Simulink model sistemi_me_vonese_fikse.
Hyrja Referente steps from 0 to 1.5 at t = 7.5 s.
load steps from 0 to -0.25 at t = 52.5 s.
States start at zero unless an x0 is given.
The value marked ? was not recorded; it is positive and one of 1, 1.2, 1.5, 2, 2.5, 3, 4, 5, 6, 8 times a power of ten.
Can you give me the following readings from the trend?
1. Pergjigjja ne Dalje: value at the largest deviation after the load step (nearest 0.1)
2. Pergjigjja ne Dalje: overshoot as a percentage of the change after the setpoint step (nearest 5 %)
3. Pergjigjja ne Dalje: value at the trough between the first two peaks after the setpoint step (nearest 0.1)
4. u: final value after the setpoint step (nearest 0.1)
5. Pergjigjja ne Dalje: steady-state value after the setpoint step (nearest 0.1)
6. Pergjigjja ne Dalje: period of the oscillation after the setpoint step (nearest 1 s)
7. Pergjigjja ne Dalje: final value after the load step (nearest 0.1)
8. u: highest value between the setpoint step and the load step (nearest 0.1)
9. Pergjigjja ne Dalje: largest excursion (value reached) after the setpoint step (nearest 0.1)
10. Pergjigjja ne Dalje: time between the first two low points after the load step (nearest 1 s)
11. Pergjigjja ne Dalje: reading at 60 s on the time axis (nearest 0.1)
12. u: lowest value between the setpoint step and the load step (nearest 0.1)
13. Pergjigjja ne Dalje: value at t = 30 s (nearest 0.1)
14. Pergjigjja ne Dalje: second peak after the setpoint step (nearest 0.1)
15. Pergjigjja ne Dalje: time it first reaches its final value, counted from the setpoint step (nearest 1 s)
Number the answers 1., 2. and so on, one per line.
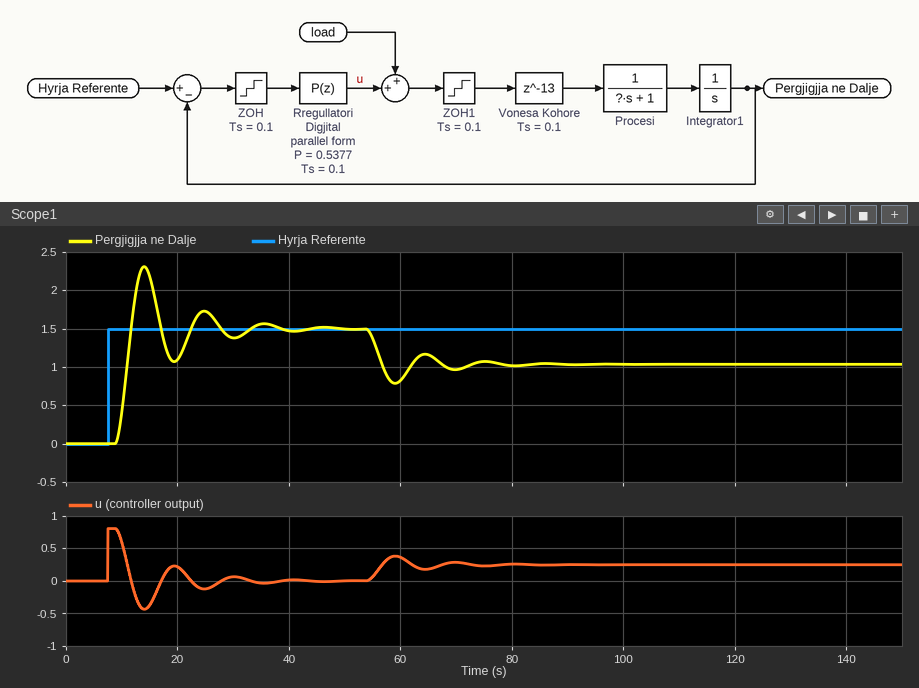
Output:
1. 0.8
2. 55 %
3. 1.1
4. 0.0
5. 1.5
6. 11 s
7. 1.0
8. 0.8
9. 2.3
10. 11 s
11. 0.8
12. -0.4
13. 1.4
14. 1.7
15. 4 s
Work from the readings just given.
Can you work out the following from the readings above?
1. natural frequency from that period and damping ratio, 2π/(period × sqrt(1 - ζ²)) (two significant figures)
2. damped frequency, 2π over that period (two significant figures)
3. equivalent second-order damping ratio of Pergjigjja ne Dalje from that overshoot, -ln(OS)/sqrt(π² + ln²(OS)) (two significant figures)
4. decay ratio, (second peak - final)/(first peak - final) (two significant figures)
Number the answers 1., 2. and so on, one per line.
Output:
1. 0.58 rad/s
2. 0.57 rad/s
3. 0.19
4. 0.25
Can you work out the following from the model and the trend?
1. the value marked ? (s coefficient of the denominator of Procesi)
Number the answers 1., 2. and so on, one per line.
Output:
1. 1
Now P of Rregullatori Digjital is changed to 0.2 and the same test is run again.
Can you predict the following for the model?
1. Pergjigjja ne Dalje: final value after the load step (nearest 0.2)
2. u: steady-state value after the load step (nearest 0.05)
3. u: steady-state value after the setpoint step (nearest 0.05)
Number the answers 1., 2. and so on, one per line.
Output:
1. 0.2
2. 0.25
3. 0.00
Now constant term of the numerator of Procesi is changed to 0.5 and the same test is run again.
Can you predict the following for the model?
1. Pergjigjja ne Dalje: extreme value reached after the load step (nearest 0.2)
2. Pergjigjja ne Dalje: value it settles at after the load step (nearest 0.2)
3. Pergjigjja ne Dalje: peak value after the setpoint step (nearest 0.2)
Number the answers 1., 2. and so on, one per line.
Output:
1. 1.0
2. 1.0
3. 1.6
